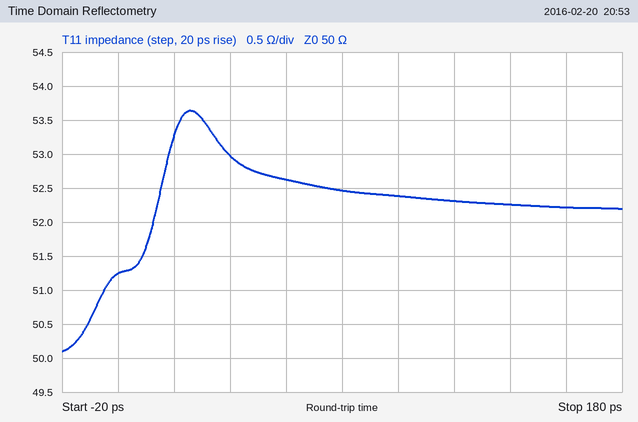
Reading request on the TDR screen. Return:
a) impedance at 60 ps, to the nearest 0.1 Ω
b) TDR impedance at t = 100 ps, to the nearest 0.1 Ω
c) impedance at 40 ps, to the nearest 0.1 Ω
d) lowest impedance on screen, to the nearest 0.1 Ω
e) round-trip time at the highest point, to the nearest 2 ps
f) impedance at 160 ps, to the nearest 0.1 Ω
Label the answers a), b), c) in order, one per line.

a) 52.6 Ω
b) 52.4 Ω
c) 53.0 Ω
d) 50.1 Ω
e) 26 ps
f) 52.2 Ω
